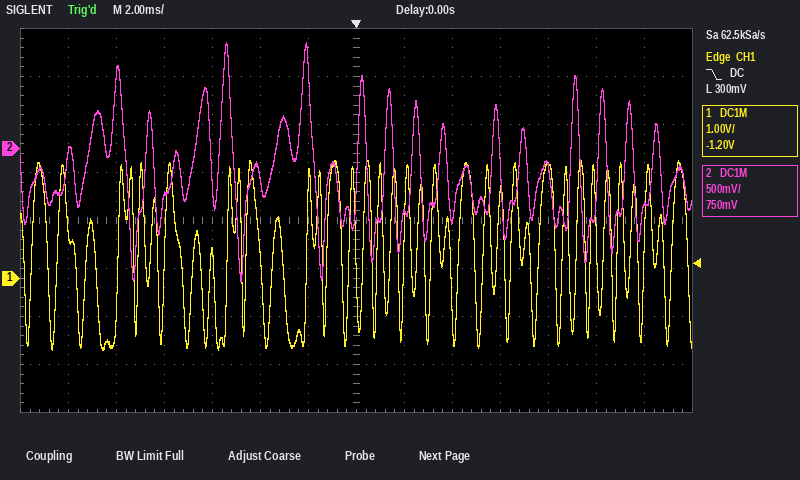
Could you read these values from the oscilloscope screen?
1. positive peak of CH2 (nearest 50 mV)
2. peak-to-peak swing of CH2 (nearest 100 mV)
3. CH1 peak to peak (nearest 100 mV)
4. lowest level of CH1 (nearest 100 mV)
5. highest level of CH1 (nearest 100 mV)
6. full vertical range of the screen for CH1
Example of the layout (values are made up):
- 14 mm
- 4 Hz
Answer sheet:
- 1.10 V
- 2.50 V
- 3.9 V
- -1.5 V
- 2.4 V
- 8 V
